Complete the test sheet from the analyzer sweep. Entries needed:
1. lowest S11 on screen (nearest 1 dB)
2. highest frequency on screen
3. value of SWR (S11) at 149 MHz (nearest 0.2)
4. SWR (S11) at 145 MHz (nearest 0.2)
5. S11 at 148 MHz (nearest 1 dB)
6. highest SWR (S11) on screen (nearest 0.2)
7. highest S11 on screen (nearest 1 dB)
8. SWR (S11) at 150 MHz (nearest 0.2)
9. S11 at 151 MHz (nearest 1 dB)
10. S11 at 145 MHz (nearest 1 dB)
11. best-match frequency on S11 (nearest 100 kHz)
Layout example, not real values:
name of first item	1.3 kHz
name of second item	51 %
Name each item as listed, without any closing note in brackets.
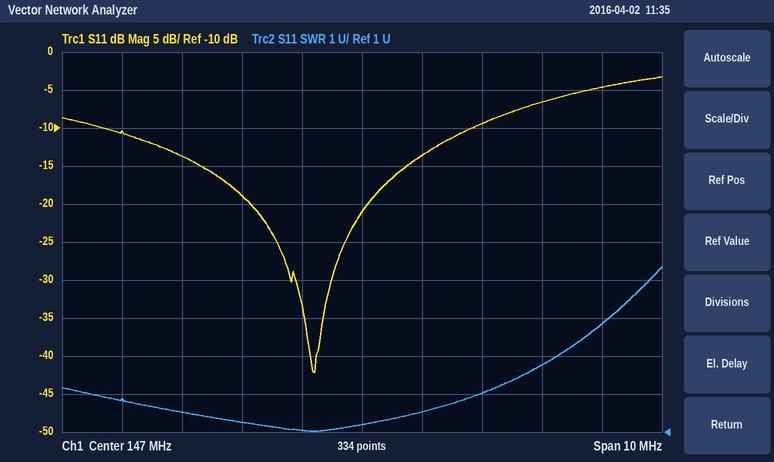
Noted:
lowest S11 on screen	-42 dB
highest frequency on screen	152 MHz
value of SWR (S11) at 149 MHz	2.0
SWR (S11) at 145 MHz	1.2
S11 at 148 MHz	-14 dB
highest SWR (S11) on screen	5.4
highest S11 on screen	-3 dB
SWR (S11) at 150 MHz	2.8
S11 at 151 MHz	-5 dB
S11 at 145 MHz	-19 dB
best-match frequency on S11	146.2 MHz
